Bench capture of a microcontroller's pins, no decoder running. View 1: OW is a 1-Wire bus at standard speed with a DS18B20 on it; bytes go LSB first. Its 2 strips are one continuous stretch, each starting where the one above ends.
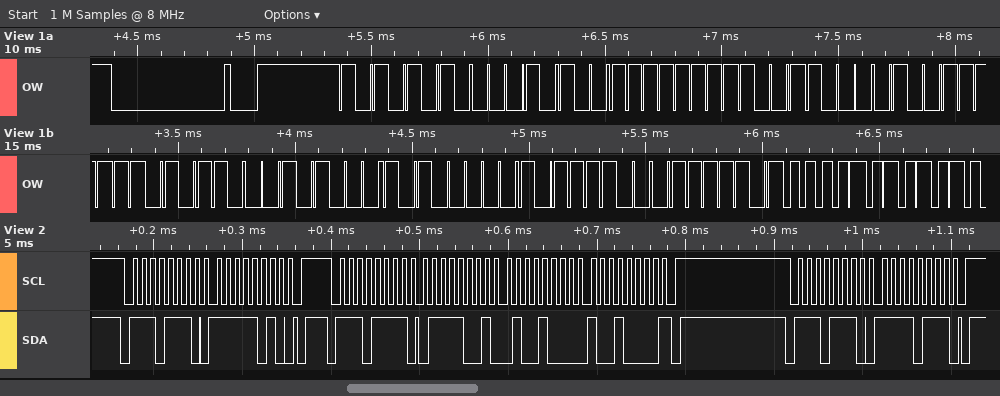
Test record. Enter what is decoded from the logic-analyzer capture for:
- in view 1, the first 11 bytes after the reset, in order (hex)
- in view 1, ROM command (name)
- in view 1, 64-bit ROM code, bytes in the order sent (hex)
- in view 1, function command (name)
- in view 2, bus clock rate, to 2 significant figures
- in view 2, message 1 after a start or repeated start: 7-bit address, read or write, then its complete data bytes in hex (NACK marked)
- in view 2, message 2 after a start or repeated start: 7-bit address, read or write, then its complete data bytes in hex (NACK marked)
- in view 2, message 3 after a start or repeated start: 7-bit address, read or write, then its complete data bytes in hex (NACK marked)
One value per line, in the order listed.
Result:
55 28 FF 19 F2 6B 14 05 3D BE 50
Match ROM
28 FF 19 F2 6B 14 05 3D
Read Scratchpad
100 kHz
0x77 write: FA
0x77 read: 79 48 90 NACK
0x77 write: F7
